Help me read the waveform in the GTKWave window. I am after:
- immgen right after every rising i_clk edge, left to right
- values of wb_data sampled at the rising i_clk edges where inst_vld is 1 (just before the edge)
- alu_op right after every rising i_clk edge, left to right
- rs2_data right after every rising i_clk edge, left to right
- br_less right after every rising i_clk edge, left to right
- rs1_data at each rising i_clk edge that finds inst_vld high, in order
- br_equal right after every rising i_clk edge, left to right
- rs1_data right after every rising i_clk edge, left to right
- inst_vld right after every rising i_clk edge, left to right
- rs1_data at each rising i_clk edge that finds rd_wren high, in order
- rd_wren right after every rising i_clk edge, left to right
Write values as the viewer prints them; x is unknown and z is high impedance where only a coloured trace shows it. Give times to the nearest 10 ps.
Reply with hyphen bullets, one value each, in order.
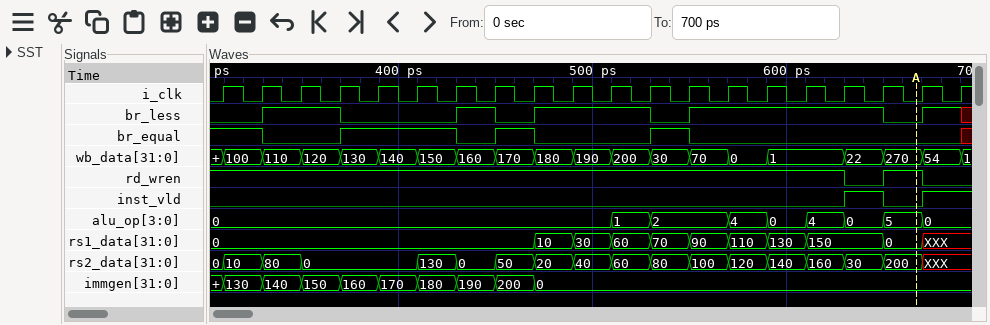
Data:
- 130, 140, 150, 160, 170, 180, 190, 200, 0, 0, 0, 0, 0, 0, 0, 0, 0, 0, 0, 0
- 22, 54
- 0, 0, 0, 0, 0, 0, 0, 0, 0, 0, 1, 2, 2, 4, 0, 4, 0, 5, 0, 0
- 10, 80, 0, 0, 0, 130, 0, 50, 20, 40, 60, 80, 100, 120, 140, 160, 30, 200, XXX, XXX
- 0 1 1 0 0 0 1 0 1 1 1 0 1 1 1 1 1 0 1 x
- 150, XXX
- 1 0 0 1 1 1 0 1 0 0 0 1 0 0 0 0 0 0 0 x
- 0, 0, 0, 0, 0, 0, 0, 0, 10, 30, 60, 70, 90, 110, 130, 150, 150, 0, XXX, XXX
- 0 0 0 0 0 0 0 0 0 0 0 0 0 0 0 0 1 0 1 1
- 0, 0, 0, 0, 0, 0, 0, 0, 0, 10, 30, 60, 70, 90, 110, 130, 150, 0
- 1 1 1 1 1 1 1 1 1 1 1 1 1 1 1 1 0 1 0 0
